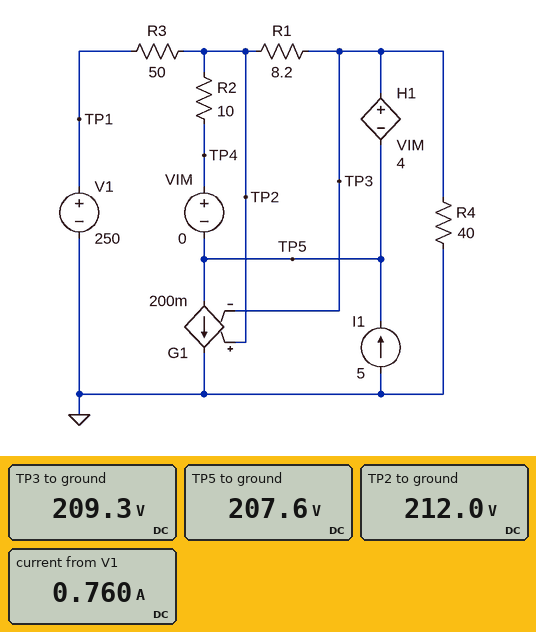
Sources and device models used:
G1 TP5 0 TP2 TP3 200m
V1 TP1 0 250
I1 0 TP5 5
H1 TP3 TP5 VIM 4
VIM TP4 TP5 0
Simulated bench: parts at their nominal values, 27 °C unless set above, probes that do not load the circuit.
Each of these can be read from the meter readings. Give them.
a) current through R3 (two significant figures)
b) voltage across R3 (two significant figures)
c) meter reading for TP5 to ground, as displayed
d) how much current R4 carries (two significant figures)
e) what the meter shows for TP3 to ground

760 mA
38 V
207.6 V
5.2 A
209.3 V
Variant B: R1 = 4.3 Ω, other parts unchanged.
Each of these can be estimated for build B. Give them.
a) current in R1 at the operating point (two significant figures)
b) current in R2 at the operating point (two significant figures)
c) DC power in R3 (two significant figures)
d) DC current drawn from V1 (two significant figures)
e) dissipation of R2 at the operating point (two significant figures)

400 mA
290 mA
24 W
690 mA
830 mW
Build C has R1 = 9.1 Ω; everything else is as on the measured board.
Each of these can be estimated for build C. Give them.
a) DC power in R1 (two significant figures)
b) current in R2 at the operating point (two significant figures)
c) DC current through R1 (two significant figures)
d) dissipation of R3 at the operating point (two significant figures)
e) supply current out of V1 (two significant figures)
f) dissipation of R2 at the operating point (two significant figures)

860 mW
470 mA
310 mA
30 W
770 mA
2.2 W
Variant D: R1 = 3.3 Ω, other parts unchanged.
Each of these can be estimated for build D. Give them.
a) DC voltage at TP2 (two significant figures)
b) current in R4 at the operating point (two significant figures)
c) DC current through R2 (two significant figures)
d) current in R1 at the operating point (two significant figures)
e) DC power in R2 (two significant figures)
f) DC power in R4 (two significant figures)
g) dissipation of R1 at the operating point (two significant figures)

220 V
5.4 A
240 mA
430 mA
560 mW
1.2 kW
610 mW
